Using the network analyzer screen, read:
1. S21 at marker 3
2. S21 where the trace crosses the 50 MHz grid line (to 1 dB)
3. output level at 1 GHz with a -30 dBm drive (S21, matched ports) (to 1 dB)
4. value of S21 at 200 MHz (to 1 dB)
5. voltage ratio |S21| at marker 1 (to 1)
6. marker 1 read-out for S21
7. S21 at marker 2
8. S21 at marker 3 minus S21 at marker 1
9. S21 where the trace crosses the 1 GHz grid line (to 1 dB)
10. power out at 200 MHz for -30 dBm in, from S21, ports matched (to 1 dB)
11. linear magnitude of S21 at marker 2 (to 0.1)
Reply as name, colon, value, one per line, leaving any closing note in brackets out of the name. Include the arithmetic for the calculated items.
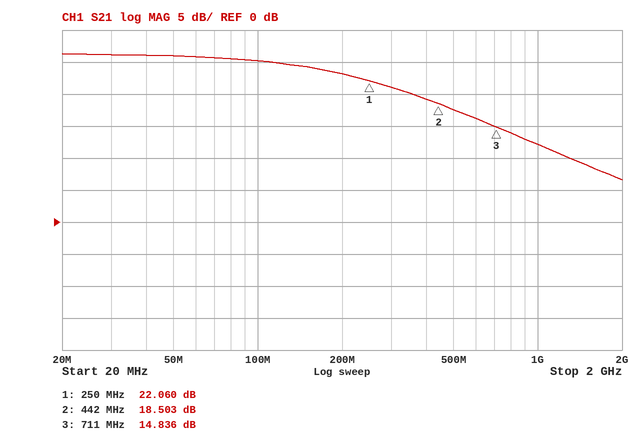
S21 at marker 3: 14.836 dB
S21 where the trace crosses the 50 MHz grid line: 26 dB
output level at 1 GHz with a -30 dBm drive (S21, matched ports): -30 dBm + (12 dB) = -18 dBm
value of S21 at 200 MHz: 23 dB
voltage ratio |S21| at marker 1: 10^(22.06/20) ≈ 13
marker 1 read-out for S21: 22.060 dB
S21 at marker 2: 18.503 dB
S21 at marker 3 minus S21 at marker 1: 14.836 − (22.06) = -7.224 dB
S21 where the trace crosses the 1 GHz grid line: 12 dB
power out at 200 MHz for -30 dBm in, from S21, ports matched: -30 dBm + (23 dB) = -7 dBm
linear magnitude of S21 at marker 2: 10^(18.503/20) ≈ 8.4
